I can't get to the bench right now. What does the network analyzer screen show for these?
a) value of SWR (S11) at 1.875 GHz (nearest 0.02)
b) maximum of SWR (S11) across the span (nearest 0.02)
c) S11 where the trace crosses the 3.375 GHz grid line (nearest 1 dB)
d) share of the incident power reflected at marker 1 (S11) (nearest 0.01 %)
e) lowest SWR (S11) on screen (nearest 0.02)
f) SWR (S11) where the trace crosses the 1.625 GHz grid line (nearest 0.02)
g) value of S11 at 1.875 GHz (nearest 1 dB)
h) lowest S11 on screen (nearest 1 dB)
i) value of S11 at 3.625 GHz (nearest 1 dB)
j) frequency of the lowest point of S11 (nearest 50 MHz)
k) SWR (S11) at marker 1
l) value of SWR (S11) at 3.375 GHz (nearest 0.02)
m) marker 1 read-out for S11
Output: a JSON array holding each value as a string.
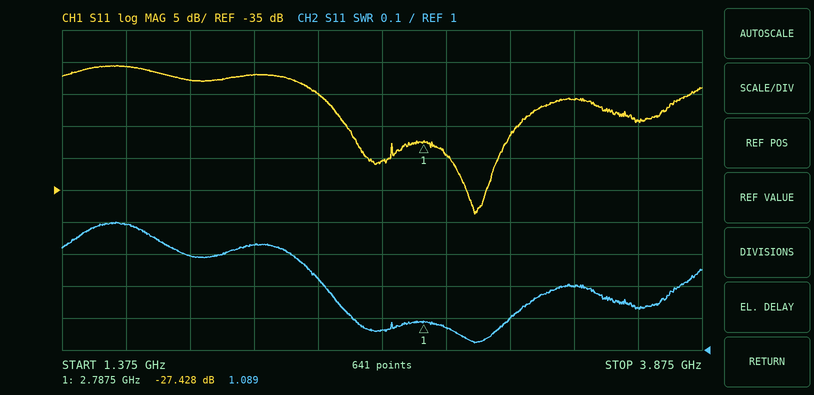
["1.30", "1.40", "-21 dB", "0.18 %", "1.02", "1.40", "-18 dB", "-39 dB", "-24 dB", "3.00 GHz", "1.089", "1.20", "-27.428 dB"]
